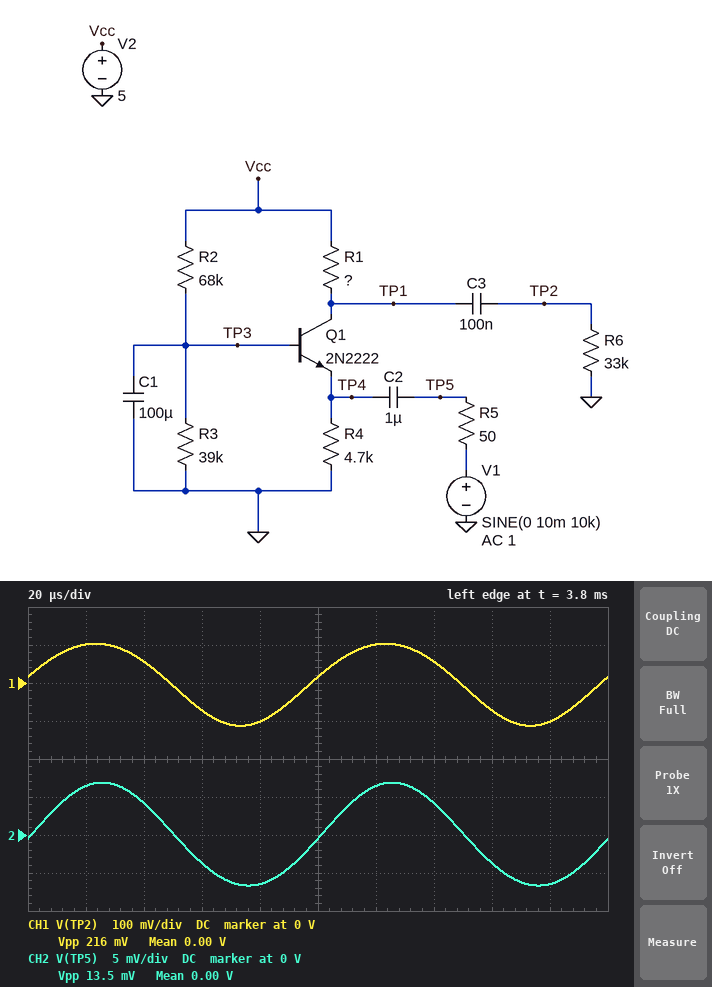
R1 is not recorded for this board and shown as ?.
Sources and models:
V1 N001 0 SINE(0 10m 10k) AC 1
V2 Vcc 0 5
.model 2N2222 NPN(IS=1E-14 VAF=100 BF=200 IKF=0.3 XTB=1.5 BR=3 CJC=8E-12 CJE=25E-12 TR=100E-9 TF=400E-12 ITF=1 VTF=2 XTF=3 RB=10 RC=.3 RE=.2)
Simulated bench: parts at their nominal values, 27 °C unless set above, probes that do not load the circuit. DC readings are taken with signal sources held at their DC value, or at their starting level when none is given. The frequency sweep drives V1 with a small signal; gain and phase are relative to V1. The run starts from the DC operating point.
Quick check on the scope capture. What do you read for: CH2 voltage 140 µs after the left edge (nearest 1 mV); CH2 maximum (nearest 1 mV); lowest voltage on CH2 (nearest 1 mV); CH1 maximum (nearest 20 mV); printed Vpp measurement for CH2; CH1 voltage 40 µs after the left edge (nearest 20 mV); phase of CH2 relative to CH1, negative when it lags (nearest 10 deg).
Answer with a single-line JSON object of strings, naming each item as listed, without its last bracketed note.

{"CH2 voltage 140 µs after the left edge": "4 mV", "CH2 maximum": "7 mV", "lowest voltage on CH2": "-7 mV", "CH1 maximum": "100 mV", "printed Vpp measurement for CH2": "13.5 mV", "CH1 voltage 40 µs after the left edge": "60 mV", "phase of CH2 relative to CH1, negative when it lags": "-10 deg"}
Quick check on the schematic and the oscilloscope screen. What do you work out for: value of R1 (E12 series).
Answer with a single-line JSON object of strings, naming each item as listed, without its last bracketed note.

{"value of R1": "1.8 kΩ"}
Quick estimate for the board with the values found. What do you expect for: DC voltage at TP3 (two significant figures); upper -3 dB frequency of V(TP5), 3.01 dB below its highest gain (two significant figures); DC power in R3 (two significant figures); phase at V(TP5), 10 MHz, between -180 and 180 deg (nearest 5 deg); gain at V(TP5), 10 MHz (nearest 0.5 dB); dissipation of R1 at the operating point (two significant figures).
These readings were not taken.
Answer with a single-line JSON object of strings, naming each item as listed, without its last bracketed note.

{"DC voltage at TP3": "1.8 V", "upper -3 dB frequency of V(TP5), 3.01 dB below its highest gain": "3.3 kHz", "DC power in R3": "82 µW", "phase at V(TP5), 10 MHz, between -180 and 180 deg": "-5 deg", "gain at V(TP5), 10 MHz": "-3.5 dB", "dissipation of R1 at the operating point": "110 µW"}
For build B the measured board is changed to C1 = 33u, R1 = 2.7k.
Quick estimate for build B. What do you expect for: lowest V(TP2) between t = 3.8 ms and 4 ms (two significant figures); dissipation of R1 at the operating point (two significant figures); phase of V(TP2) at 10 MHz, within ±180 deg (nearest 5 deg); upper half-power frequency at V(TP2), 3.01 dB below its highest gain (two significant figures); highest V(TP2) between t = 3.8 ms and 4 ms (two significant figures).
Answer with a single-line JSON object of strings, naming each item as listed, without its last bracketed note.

{"lowest V(TP2) between t = 3.8 ms and 4 ms": "-160 mV", "dissipation of R1 at the operating point": "170 µW", "phase of V(TP2) at 10 MHz, within ±180 deg": "-45 deg", "upper half-power frequency at V(TP2), 3.01 dB below its highest gain": "12 MHz", "highest V(TP2) between t = 3.8 ms and 4 ms": "150 mV"}
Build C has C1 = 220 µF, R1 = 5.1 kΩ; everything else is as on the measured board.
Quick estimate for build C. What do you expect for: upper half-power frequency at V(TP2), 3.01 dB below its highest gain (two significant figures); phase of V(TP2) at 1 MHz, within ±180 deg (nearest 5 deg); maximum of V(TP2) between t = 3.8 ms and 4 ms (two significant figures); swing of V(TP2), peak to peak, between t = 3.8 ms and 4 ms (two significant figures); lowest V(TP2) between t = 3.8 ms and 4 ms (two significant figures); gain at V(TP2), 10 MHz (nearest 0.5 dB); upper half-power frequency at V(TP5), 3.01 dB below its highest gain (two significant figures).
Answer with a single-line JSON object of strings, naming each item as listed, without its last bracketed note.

{"upper half-power frequency at V(TP2), 3.01 dB below its highest gain": "6.4 MHz", "phase of V(TP2) at 1 MHz, within ±180 deg": "-10 deg", "maximum of V(TP2) between t = 3.8 ms and 4 ms": "270 mV", "swing of V(TP2), peak to peak, between t = 3.8 ms and 4 ms": "560 mV", "lowest V(TP2) between t = 3.8 ms and 4 ms": "-290 mV", "gain at V(TP2), 10 MHz": "23.5 dB", "upper half-power frequency at V(TP5), 3.01 dB below its highest gain": "3.4 kHz"}
